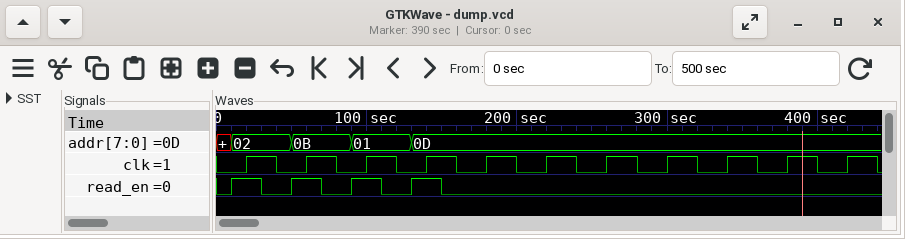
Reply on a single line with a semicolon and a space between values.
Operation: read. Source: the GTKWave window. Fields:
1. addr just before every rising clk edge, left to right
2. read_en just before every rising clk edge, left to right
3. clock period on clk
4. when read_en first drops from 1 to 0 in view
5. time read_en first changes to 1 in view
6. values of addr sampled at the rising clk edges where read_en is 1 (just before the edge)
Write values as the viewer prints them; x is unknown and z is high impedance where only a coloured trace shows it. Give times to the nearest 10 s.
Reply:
02, 0B, 01, 0D, 0D, 0D, 0D, 0D, 0D, 0D, 0D; 1 1 1 1 0 0 0 0 0 0 0; 40 s; 30 s; 10 s; 02, 0B, 01, 0D
